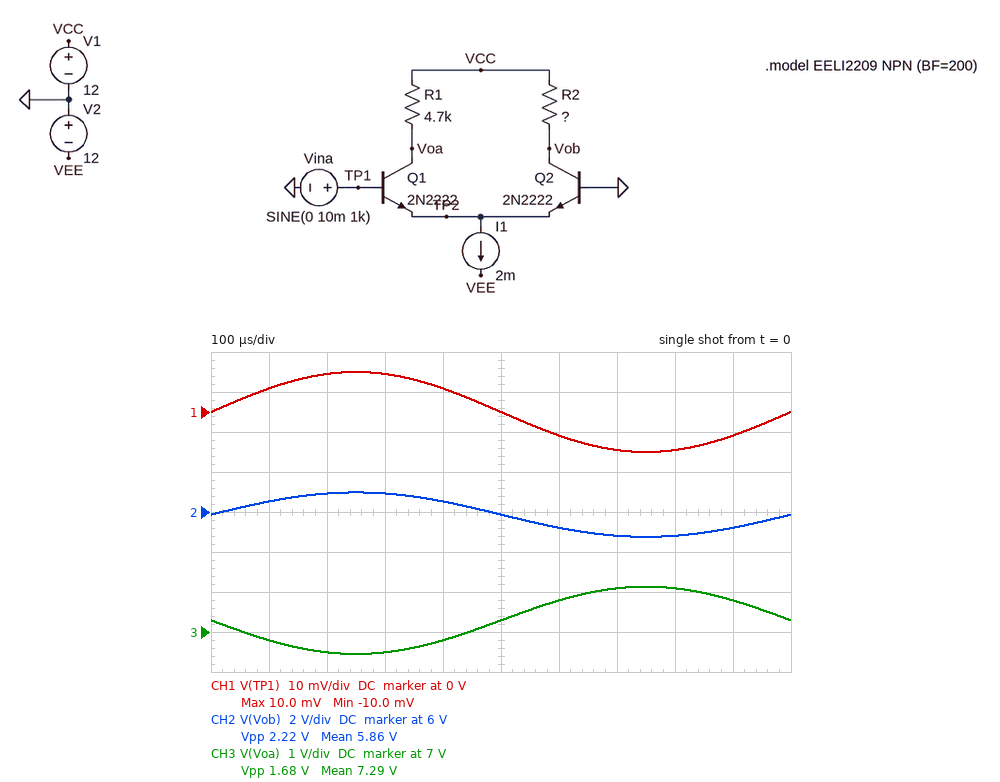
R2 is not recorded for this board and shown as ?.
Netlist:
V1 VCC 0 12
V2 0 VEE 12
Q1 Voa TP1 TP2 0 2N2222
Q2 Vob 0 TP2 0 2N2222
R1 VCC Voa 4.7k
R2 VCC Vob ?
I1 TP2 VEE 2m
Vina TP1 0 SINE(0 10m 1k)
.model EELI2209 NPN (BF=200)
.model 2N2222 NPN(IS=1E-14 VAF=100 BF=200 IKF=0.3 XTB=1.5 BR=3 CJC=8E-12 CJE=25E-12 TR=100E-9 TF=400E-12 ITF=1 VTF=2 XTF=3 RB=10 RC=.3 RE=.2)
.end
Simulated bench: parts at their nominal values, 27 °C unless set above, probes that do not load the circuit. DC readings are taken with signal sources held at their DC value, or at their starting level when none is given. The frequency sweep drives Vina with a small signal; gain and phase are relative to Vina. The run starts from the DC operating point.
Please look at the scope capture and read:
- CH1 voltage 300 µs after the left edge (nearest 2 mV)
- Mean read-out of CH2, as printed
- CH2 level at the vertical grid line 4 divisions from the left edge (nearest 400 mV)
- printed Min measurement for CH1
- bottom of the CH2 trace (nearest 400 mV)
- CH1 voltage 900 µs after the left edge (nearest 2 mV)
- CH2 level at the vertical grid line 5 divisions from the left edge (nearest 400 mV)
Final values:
10 mV
5.86 V
6.4 V
-10.0 mV
4.8 V
-6 mV
6.0 V
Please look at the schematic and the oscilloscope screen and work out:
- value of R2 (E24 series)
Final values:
6.2 kΩ
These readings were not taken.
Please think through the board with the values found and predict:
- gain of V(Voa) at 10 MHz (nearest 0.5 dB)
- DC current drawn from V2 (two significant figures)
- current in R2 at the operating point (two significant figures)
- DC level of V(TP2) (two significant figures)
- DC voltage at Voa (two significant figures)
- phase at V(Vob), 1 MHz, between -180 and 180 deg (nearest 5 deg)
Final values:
33.5 dB
2.0 mA
990 µA
-650 mV
7.3 V
-10 deg
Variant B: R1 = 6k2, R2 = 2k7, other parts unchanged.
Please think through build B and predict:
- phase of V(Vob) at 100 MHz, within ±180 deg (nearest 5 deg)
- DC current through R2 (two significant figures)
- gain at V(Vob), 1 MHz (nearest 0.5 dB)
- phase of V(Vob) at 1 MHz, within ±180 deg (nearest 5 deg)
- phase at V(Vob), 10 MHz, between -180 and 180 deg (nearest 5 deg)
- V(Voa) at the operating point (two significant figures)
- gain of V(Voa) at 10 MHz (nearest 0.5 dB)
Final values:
-95 deg
1.0 mA
34.0 dB
-5 deg
-40 deg
5.9 V
34.5 dB
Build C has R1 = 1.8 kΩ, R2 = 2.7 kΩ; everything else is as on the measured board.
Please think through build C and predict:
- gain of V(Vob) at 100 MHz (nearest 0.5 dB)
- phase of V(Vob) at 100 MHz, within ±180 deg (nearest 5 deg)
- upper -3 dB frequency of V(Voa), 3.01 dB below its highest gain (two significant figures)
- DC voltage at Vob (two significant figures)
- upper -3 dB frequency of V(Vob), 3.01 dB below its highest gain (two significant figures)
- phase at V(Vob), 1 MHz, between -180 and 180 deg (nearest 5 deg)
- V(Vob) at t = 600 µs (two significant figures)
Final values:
15.5 dB
-95 deg
18 MHz
9.3 V
13 MHz
-5 deg
9.0 V
